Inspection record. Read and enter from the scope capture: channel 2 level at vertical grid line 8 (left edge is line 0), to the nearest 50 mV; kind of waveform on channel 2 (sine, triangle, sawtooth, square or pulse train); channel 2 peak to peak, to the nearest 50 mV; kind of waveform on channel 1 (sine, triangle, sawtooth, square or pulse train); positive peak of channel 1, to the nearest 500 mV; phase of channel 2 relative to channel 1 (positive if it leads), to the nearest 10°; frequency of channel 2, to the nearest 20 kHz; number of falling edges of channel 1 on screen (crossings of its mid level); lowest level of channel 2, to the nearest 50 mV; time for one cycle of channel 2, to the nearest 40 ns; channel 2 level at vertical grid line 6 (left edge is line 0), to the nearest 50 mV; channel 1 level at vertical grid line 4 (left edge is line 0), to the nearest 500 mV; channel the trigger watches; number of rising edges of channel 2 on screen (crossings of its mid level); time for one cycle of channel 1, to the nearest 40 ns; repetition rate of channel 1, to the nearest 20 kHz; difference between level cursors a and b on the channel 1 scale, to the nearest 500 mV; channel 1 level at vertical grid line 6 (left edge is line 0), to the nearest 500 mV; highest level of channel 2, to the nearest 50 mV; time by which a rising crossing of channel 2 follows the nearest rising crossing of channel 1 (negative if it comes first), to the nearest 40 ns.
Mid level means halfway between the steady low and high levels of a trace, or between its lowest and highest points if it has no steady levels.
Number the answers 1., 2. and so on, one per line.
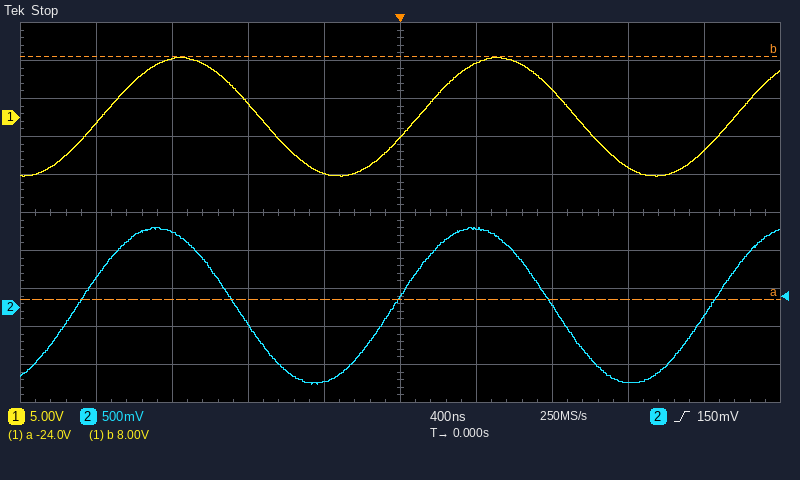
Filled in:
1. -1.00 V
2. sine
3. 2.05 V
4. sine
5. 8.0 V
6. +30°
7. 600 kHz
8. 2
9. -1.00 V
10. 1.68 µs
11. 1.05 V
12. -7.5 V
13. channel 2
14. 3
15. 1.68 µs
16. 600 kHz
17. 32.0 V
18. 7.0 V
19. 1.05 V
20. -120 ns
